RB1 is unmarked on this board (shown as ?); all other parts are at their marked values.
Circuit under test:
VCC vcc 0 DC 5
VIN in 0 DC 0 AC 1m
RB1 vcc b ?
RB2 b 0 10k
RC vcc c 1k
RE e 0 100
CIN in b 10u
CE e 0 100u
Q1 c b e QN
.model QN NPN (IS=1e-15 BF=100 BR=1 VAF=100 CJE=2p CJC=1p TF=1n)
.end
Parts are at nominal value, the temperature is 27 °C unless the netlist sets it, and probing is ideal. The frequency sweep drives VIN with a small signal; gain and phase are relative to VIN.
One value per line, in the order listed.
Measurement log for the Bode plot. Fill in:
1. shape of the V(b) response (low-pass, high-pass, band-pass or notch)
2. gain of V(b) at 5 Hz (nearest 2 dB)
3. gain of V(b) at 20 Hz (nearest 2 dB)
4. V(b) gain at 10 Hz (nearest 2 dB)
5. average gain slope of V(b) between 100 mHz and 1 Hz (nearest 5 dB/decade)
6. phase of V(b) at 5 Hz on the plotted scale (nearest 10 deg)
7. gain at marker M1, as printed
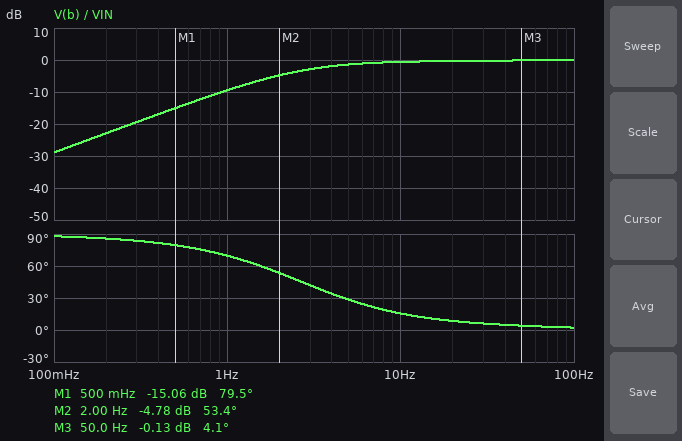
high-pass
-2 dB
0 dB
0 dB
20 dB/decade
30 deg
-15.06 dB
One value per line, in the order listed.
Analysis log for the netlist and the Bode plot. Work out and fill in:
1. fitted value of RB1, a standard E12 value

56 kΩ
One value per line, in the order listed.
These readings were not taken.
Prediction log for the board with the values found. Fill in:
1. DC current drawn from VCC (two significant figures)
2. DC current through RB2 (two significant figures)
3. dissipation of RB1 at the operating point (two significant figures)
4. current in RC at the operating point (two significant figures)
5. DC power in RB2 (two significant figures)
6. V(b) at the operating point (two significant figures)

450 µA
73 µA
330 µW
380 µA
53 µW
730 mV
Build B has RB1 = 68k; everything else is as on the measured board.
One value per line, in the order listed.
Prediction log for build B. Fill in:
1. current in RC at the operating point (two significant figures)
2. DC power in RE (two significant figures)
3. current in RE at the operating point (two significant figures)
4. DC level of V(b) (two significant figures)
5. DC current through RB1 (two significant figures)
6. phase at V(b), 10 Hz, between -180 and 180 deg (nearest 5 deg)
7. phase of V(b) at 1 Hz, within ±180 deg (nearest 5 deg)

44 µA
200 nW
45 µA
640 mV
64 µA
10 deg
65 deg
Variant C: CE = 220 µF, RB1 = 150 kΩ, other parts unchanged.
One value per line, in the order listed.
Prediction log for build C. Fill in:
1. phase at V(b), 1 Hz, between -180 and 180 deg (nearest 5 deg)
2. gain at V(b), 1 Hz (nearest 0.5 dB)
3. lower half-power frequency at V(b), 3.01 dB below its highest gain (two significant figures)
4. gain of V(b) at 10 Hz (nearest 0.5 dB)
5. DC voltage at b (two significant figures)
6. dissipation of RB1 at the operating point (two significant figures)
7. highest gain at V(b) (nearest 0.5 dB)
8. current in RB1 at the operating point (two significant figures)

60 deg
-6.0 dB
1.7 Hz
0 dB
310 mV
150 µW
0 dB
31 µA
